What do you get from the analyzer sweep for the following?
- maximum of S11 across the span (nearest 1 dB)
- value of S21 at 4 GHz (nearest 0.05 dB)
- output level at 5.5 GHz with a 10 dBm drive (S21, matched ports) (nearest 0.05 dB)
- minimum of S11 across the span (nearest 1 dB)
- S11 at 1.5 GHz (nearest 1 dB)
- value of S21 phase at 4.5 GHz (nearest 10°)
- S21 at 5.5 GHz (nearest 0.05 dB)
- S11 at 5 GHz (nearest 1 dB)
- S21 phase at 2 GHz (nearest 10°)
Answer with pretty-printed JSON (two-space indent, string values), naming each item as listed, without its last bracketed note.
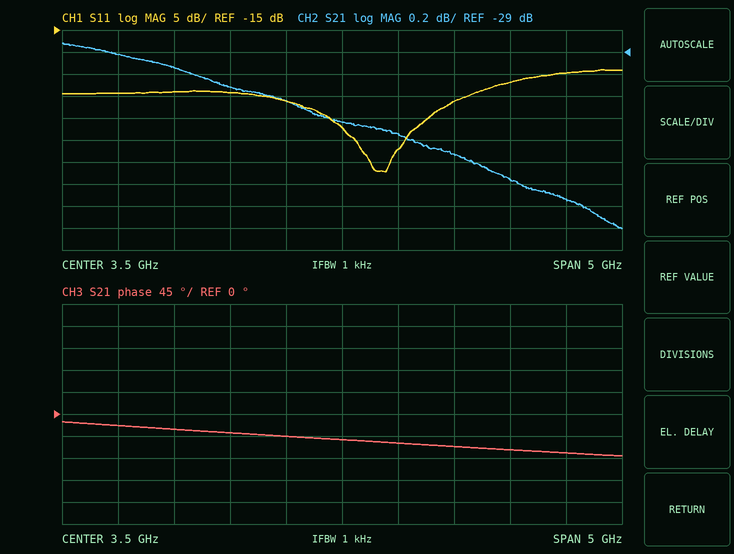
{
  "maximum of S11 across the span": "-24 dB",
  "value of S21 at 4 GHz": "-29.75 dB",
  "output level at 5.5 GHz with a 10 dBm drive (S21, matched ports)": "-20.35 dBm",
  "minimum of S11 across the span": "-47 dB",
  "S11 at 1.5 GHz": "-29 dB",
  "value of S21 phase at 4.5 GHz": "-70°",
  "S21 at 5.5 GHz": "-30.35 dB",
  "S11 at 5 GHz": "-27 dB",
  "S21 phase at 2 GHz": "-30°"
}
